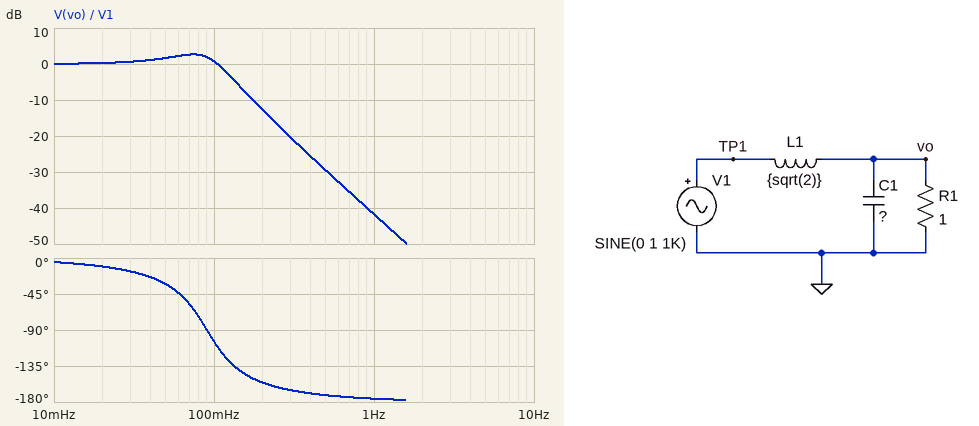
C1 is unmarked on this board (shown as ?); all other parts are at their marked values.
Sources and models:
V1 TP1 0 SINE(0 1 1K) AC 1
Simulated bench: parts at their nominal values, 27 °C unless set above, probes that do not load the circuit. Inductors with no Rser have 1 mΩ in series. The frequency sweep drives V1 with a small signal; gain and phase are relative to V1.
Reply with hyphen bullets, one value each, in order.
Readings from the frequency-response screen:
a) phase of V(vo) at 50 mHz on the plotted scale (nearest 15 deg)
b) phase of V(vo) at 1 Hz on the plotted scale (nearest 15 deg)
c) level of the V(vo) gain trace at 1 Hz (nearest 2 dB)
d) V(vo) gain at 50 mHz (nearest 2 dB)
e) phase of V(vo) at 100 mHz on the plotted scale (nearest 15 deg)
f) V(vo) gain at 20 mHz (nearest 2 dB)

- -30 deg
- -180 deg
- -42 dB
- 2 dB
- -105 deg
- 0 dB
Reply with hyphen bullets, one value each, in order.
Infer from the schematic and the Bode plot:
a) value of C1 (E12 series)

- 2.2 F
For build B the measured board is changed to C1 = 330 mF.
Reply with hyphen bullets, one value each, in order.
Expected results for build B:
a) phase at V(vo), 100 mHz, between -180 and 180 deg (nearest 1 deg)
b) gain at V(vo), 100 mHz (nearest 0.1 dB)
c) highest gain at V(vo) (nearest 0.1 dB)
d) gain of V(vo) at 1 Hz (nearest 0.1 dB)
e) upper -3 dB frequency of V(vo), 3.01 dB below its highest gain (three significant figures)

- -47 deg
- -1.6 dB
- 0 dB
- -25.8 dB
- 143 mHz
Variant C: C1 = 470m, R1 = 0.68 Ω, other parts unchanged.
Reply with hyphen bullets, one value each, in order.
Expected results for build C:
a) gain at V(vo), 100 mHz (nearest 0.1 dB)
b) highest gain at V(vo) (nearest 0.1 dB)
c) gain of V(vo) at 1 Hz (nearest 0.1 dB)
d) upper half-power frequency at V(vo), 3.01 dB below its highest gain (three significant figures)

- -3.5 dB
- 0 dB
- -29.1 dB
- 90.0 mHz
